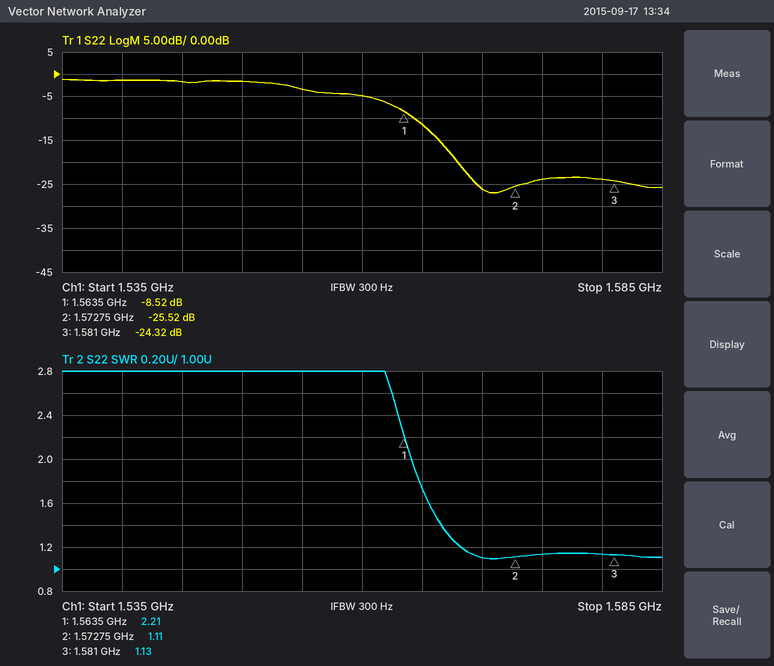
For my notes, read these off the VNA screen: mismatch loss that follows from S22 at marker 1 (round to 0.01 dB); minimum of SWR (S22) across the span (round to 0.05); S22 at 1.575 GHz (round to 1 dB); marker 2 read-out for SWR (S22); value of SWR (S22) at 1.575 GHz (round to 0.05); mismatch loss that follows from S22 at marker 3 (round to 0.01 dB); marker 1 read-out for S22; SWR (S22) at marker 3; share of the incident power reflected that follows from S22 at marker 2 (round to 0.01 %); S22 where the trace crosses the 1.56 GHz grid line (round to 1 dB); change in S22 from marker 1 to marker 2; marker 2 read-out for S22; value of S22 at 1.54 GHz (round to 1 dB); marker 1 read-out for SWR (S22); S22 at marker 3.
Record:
0.66 dB
1.10
-24 dB
1.11
1.15
0.02 dB
-8.52 dB
1.13
0.28 %
-5 dB
-17.00 dB
-25.52 dB
-1 dB
2.21
-24.32 dB
